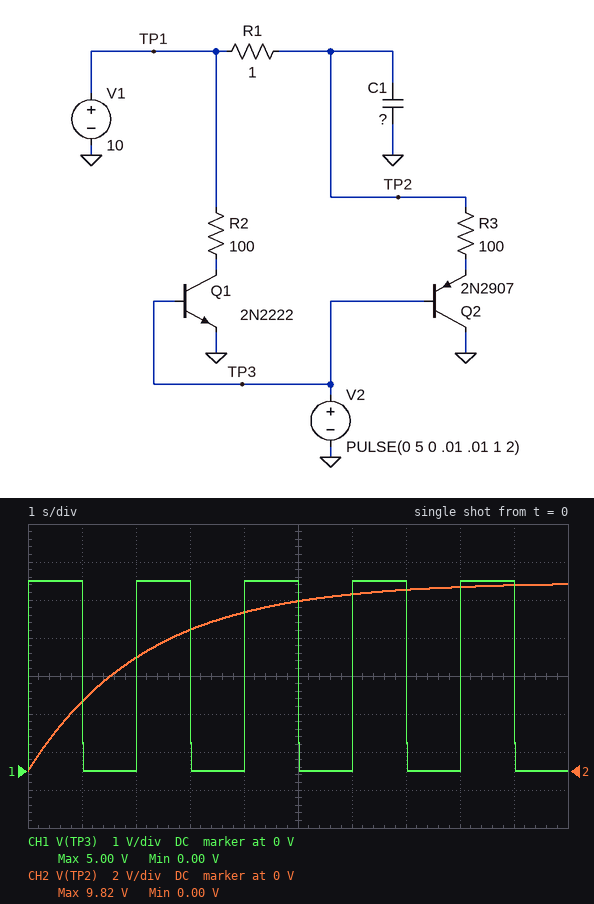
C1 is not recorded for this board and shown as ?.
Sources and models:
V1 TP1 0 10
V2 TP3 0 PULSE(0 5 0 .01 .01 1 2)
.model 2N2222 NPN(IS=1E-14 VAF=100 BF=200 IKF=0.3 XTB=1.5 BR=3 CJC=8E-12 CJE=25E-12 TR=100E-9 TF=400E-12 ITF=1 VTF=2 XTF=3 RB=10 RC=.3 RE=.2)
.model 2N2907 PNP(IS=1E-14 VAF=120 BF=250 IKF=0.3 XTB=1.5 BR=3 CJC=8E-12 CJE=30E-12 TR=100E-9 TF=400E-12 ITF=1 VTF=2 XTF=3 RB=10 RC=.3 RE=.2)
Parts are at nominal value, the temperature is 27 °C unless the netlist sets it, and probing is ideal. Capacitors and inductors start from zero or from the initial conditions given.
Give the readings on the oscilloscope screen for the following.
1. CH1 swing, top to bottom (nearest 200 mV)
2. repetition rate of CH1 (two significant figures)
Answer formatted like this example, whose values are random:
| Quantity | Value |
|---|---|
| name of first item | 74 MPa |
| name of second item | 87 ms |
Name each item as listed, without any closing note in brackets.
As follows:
| Quantity | Value |
|---|---|
| CH1 swing, top to bottom | 5.0 V |
| repetition rate of CH1 | 500 mHz |
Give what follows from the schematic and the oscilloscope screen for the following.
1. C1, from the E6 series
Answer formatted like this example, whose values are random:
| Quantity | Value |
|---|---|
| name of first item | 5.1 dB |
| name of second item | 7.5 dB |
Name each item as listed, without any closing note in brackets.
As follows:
| Quantity | Value |
|---|---|
| C1, from the E6 series | 2.2 F |
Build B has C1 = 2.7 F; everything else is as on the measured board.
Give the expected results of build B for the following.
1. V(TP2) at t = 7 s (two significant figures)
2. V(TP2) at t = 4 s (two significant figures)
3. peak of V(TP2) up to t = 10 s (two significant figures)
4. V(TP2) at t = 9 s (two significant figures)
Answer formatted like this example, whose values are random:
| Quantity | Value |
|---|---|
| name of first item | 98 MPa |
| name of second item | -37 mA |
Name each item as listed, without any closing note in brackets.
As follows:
| Quantity | Value |
|---|---|
| V(TP2) at t = 7 s | 9.2 V |
| V(TP2) at t = 4 s | 7.7 V |
| peak of V(TP2) up to t = 10 s | 9.7 V |
| V(TP2) at t = 9 s | 9.6 V |
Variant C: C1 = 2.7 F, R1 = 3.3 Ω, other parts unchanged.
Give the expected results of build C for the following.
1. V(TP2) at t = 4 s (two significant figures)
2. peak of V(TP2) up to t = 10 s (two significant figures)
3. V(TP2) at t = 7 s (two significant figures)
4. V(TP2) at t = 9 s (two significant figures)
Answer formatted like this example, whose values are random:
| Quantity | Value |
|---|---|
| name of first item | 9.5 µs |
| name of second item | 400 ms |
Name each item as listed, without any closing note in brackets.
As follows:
| Quantity | Value |
|---|---|
| V(TP2) at t = 4 s | 3.6 V |
| peak of V(TP2) up to t = 10 s | 6.7 V |
| V(TP2) at t = 7 s | 5.4 V |
| V(TP2) at t = 9 s | 6.3 V |
